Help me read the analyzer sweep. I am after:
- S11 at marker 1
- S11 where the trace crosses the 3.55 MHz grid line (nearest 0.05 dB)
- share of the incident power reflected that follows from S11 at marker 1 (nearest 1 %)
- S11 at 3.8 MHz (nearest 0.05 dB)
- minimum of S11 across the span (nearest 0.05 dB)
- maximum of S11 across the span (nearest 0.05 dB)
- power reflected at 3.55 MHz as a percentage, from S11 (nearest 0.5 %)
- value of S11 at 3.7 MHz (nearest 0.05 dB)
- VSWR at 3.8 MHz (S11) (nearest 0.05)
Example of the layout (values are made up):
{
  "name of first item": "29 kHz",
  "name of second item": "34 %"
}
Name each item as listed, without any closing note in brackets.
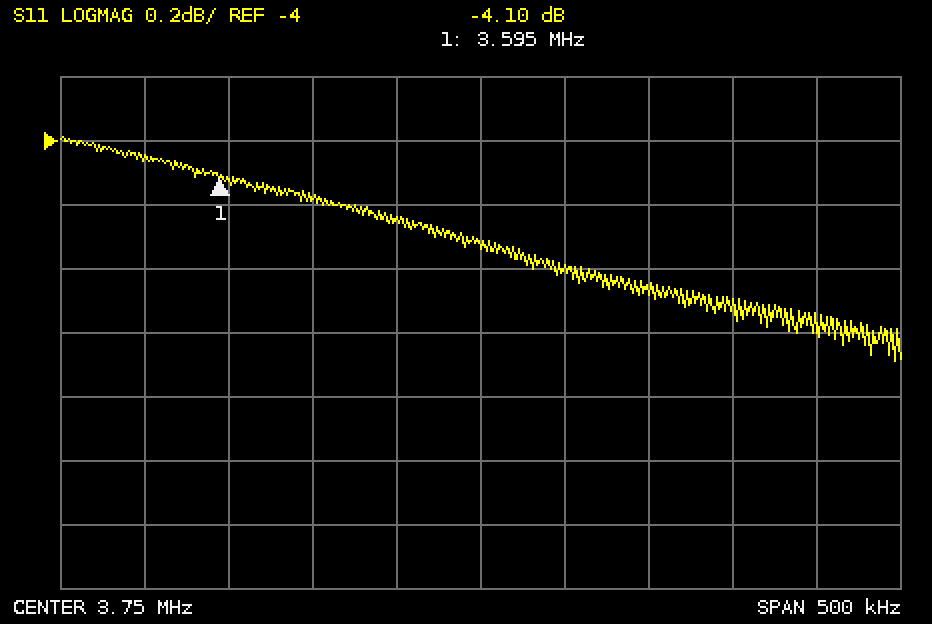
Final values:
{
  "S11 at marker 1": "-4.10 dB",
  "S11 where the trace crosses the 3.55 MHz grid line": "-4.05 dB",
  "share of the incident power reflected that follows from S11 at marker 1": "39 %",
  "S11 at 3.8 MHz": "-4.40 dB",
  "minimum of S11 across the span": "-4.70 dB",
  "maximum of S11 across the span": "-4.00 dB",
  "power reflected at 3.55 MHz as a percentage, from S11": "39.5 %",
  "value of S11 at 3.7 MHz": "-4.25 dB",
  "VSWR at 3.8 MHz (S11)": "4.05"
}
